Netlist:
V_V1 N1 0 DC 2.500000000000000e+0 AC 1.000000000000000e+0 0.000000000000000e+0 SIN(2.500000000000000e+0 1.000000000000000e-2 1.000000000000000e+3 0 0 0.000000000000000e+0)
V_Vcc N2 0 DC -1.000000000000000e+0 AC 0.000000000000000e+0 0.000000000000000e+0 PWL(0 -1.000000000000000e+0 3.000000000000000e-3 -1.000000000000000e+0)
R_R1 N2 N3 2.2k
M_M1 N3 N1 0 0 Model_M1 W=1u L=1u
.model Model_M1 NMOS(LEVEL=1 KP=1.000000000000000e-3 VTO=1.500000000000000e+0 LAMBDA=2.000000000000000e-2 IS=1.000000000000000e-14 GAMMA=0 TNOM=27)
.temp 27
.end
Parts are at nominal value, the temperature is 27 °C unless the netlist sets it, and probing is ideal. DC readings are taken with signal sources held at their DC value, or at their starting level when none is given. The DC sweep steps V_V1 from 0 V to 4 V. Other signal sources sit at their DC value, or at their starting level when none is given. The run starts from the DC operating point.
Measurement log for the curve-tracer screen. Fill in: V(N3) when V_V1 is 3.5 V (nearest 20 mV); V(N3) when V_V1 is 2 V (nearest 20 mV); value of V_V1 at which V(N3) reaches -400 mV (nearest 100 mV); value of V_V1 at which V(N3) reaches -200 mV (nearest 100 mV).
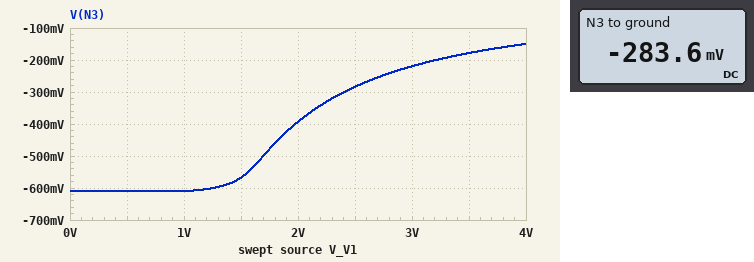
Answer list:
-180 mV
-400 mV
2.0 V
3.2 V
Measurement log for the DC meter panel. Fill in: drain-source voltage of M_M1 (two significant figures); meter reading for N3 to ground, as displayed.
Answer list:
-280 mV
-283.6 mV
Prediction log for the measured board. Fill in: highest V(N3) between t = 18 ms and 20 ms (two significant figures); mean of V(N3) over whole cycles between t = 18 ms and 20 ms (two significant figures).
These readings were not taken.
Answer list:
-280 mV
-280 mV
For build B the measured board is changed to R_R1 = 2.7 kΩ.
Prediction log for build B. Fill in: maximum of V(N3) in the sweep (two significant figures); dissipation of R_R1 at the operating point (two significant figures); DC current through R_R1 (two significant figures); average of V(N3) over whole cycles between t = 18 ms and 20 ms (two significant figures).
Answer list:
-130 mV
210 µW
280 µA
-250 mV
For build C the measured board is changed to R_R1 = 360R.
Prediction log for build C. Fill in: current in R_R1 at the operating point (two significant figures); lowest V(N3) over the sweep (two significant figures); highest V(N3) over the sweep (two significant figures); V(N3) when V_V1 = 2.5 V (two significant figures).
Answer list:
1.1 mA
-650 mV
-500 mV
-620 mV
